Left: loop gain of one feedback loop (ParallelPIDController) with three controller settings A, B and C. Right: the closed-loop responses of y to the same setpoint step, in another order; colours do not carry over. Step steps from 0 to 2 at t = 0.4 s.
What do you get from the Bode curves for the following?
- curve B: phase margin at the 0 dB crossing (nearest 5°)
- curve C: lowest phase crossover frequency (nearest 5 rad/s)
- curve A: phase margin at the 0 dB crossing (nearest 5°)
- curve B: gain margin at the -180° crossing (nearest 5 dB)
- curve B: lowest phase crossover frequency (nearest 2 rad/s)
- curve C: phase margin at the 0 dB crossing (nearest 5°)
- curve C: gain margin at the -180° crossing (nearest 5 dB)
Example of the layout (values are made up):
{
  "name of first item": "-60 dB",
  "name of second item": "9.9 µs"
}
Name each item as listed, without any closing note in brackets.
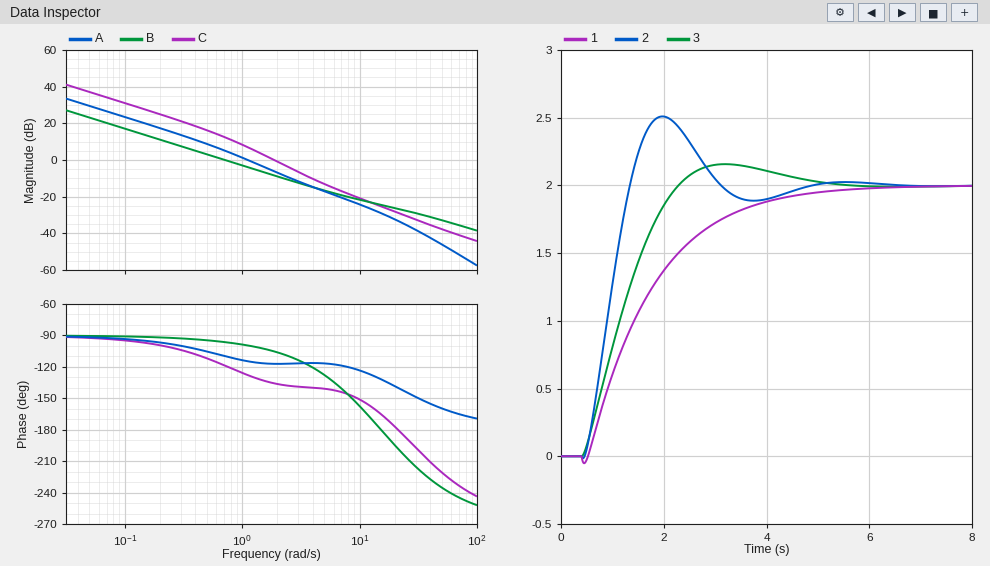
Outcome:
{
  "curve B: phase margin at the 0 dB crossing": "85°",
  "curve C: lowest phase crossover frequency": "20 rad/s",
  "curve A: phase margin at the 0 dB crossing": "65°",
  "curve B: gain margin at the -180° crossing": "25 dB",
  "curve B: lowest phase crossover frequency": "16 rad/s",
  "curve C: phase margin at the 0 dB crossing": "45°",
  "curve C: gain margin at the -180° crossing": "30 dB"
}
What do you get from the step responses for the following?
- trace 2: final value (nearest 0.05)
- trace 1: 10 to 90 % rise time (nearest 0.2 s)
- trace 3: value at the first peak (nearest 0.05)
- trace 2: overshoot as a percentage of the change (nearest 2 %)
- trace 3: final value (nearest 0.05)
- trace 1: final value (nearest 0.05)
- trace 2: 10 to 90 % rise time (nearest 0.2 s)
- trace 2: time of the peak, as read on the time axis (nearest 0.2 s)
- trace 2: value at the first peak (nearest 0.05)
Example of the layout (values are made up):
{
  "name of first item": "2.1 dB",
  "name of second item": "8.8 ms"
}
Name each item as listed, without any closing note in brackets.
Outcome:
{
  "trace 2: final value": "2.00",
  "trace 1: 10 to 90 % rise time": "2.8 s",
  "trace 3: value at the first peak": "2.15",
  "trace 2: overshoot as a percentage of the change": "26 %",
  "trace 3: final value": "2.00",
  "trace 1: final value": "2.00",
  "trace 2: 10 to 90 % rise time": "0.6 s",
  "trace 2: time of the peak, as read on the time axis": "2.0 s",
  "trace 2: value at the first peak": "2.50"
}
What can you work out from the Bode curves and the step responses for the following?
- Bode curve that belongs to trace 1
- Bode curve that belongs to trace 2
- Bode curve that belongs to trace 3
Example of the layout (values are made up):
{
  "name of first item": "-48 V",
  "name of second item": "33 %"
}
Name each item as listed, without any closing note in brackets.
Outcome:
{
  "Bode curve that belongs to trace 1": "B",
  "Bode curve that belongs to trace 2": "C",
  "Bode curve that belongs to trace 3": "A"
}
